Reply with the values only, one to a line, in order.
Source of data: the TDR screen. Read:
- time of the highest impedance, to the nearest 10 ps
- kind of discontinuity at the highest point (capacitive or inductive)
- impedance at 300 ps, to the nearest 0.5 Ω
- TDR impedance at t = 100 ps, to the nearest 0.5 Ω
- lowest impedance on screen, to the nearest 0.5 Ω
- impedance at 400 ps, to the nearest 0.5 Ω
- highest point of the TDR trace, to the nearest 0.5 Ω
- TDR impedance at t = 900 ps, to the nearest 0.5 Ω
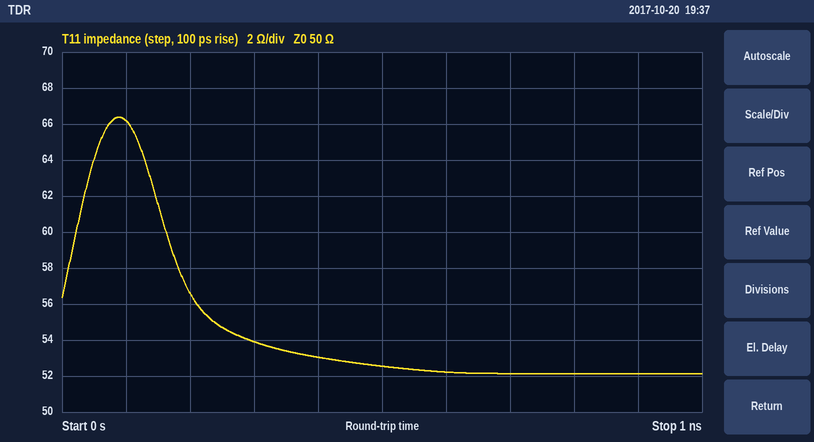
90 ps
inductive
54.0 Ω
66.0 Ω
52.0 Ω
53.0 Ω
66.5 Ω
52.0 Ω
